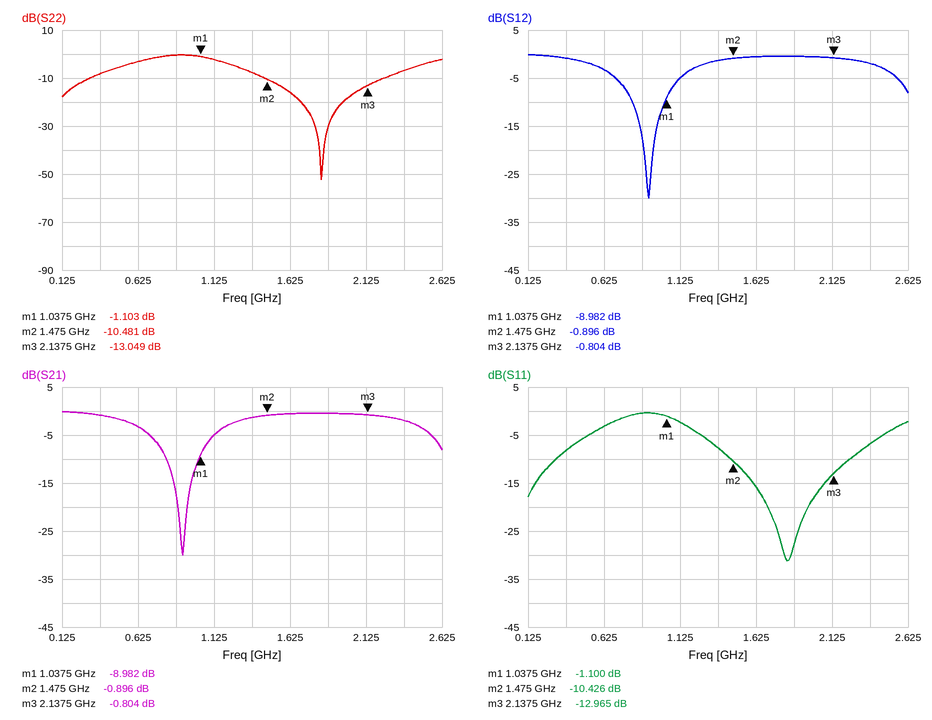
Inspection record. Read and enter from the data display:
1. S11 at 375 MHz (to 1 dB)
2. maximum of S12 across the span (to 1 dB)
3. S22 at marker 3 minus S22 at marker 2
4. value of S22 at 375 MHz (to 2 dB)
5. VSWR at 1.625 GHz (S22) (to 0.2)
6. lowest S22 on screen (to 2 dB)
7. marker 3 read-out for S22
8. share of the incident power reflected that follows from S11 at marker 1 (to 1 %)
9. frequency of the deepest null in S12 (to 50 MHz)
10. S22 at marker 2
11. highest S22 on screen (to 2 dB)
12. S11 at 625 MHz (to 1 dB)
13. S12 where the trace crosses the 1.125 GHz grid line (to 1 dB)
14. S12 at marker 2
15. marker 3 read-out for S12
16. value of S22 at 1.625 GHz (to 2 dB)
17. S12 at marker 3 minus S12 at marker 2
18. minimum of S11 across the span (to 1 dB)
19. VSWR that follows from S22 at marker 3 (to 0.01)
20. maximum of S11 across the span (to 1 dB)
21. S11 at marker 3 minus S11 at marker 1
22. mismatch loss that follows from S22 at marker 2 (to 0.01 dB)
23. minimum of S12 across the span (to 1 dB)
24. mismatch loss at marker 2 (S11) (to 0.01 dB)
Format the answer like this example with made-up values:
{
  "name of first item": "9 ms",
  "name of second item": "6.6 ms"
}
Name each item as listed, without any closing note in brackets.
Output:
{
  "S11 at 375 MHz": "-8 dB",
  "maximum of S12 across the span": "0 dB",
  "S22 at marker 3 minus S22 at marker 2": "-2.568 dB",
  "value of S22 at 375 MHz": "-8 dB",
  "VSWR at 1.625 GHz (S22)": "1.4",
  "lowest S22 on screen": "-52 dB",
  "marker 3 read-out for S22": "-13.049 dB",
  "share of the incident power reflected that follows from S11 at marker 1": "78 %",
  "frequency of the deepest null in S12": "900 MHz",
  "S22 at marker 2": "-10.481 dB",
  "highest S22 on screen": "0 dB",
  "S11 at 625 MHz": "-3 dB",
  "S12 where the trace crosses the 1.125 GHz grid line": "-5 dB",
  "S12 at marker 2": "-0.896 dB",
  "marker 3 read-out for S12": "-0.804 dB",
  "value of S22 at 1.625 GHz": "-16 dB",
  "S12 at marker 3 minus S12 at marker 2": "0.092 dB",
  "minimum of S11 across the span": "-31 dB",
  "VSWR that follows from S22 at marker 3": "1.57",
  "maximum of S11 across the span": "0 dB",
  "S11 at marker 3 minus S11 at marker 1": "-11.865 dB",
  "mismatch loss that follows from S22 at marker 2": "0.41 dB",
  "minimum of S12 across the span": "-30 dB",
  "mismatch loss at marker 2 (S11)": "0.41 dB"
}
